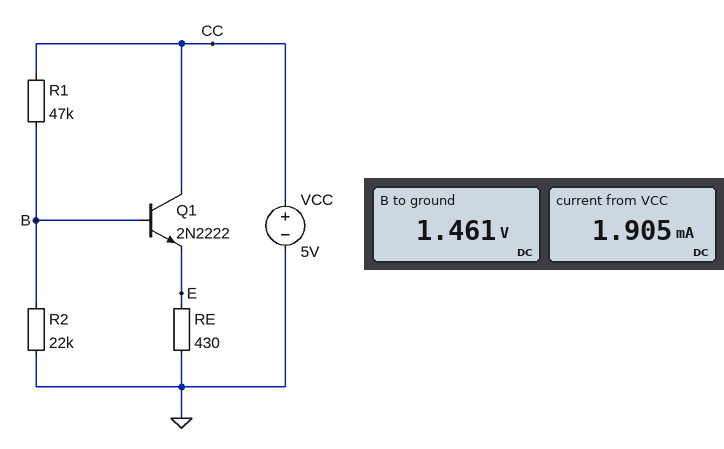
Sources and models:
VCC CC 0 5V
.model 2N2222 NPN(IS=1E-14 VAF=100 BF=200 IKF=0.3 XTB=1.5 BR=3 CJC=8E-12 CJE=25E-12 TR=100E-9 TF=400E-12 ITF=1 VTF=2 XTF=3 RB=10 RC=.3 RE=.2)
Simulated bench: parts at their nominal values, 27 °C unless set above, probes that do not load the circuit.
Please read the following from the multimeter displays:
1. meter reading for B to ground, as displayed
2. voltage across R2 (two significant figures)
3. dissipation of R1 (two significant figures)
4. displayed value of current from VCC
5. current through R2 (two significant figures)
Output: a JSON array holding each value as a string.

["1.461 V", "1.5 V", "270 µW", "1.905 mA", "66 µA"]
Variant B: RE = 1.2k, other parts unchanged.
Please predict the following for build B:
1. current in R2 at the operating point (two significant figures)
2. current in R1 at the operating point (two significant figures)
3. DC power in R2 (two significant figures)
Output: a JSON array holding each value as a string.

["70 µA", "74 µA", "110 µW"]
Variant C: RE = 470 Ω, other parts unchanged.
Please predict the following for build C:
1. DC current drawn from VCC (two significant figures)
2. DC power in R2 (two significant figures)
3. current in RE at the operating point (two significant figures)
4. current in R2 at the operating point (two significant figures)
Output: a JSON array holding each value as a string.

["1.8 mA", "98 µW", "1.7 mA", "67 µA"]
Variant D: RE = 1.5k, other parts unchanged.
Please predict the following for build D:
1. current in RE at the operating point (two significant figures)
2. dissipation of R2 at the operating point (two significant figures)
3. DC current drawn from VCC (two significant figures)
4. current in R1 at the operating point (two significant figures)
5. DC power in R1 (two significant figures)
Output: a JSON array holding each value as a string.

["610 µA", "110 µW", "680 µA", "73 µA", "250 µW"]
